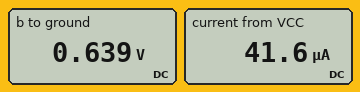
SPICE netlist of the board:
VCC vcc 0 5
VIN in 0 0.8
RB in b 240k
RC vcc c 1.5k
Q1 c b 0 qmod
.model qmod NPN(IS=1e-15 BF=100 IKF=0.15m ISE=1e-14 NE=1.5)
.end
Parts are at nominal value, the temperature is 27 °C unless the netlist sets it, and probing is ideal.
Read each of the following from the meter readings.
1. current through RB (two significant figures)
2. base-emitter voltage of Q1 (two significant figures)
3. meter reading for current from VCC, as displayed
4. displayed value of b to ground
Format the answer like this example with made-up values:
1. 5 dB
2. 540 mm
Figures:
1. 670 nA
2. 640 mV
3. 41.6 µA
4. 0.639 V
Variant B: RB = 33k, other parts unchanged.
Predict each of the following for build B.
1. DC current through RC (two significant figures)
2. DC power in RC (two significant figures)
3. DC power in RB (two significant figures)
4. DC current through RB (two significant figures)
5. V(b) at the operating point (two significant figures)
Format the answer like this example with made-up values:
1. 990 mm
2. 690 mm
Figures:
1. 150 µA
2. 35 µW
3. 410 nW
4. 3.5 µA
5. 680 mV
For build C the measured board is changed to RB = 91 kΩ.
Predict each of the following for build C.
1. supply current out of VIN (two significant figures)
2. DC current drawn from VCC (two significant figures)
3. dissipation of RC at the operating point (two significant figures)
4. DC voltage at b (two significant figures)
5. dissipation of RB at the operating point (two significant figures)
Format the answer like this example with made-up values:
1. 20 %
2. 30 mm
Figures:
1. 1.5 µA
2. 82 µA
3. 10 µW
4. 660 mV
5. 210 nW
